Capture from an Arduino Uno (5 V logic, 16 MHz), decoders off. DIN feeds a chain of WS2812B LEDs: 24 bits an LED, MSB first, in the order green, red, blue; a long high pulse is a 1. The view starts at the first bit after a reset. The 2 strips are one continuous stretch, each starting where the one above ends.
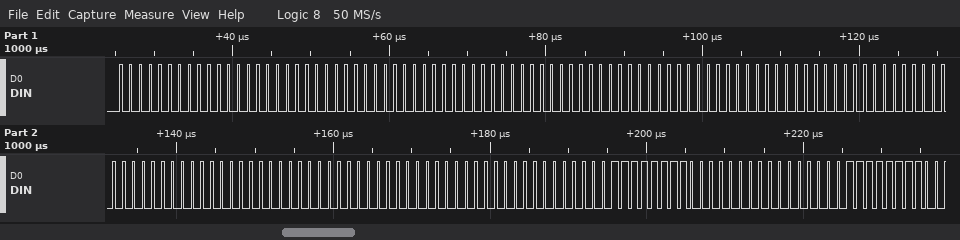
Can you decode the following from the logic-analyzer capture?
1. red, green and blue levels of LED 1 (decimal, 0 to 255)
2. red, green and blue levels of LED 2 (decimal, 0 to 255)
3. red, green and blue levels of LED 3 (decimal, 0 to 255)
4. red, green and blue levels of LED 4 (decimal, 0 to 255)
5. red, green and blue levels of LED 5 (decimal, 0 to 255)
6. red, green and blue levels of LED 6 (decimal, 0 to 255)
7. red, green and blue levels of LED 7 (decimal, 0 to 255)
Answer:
0, 0, 0
0, 0, 0
0, 0, 0
0, 0, 0
0, 0, 0
0, 0, 255
0, 0, 255
